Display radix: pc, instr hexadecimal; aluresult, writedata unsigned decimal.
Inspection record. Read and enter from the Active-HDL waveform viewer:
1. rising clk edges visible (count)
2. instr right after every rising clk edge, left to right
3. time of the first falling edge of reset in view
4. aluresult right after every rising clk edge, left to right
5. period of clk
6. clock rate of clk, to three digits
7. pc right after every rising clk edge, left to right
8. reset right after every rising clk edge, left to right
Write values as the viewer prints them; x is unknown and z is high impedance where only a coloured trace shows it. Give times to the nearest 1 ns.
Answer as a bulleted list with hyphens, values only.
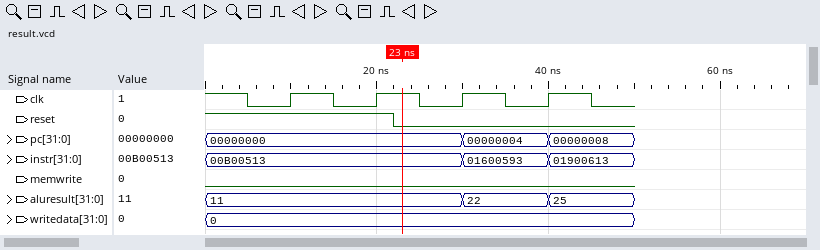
- 4
- 00B00513, 00B00513, 01600593, 01900613
- 22 ns
- 11, 11, 22, 25
- 10 ns
- 100 MHz
- 00000000, 00000000, 00000004, 00000008
- 1 1 0 0
